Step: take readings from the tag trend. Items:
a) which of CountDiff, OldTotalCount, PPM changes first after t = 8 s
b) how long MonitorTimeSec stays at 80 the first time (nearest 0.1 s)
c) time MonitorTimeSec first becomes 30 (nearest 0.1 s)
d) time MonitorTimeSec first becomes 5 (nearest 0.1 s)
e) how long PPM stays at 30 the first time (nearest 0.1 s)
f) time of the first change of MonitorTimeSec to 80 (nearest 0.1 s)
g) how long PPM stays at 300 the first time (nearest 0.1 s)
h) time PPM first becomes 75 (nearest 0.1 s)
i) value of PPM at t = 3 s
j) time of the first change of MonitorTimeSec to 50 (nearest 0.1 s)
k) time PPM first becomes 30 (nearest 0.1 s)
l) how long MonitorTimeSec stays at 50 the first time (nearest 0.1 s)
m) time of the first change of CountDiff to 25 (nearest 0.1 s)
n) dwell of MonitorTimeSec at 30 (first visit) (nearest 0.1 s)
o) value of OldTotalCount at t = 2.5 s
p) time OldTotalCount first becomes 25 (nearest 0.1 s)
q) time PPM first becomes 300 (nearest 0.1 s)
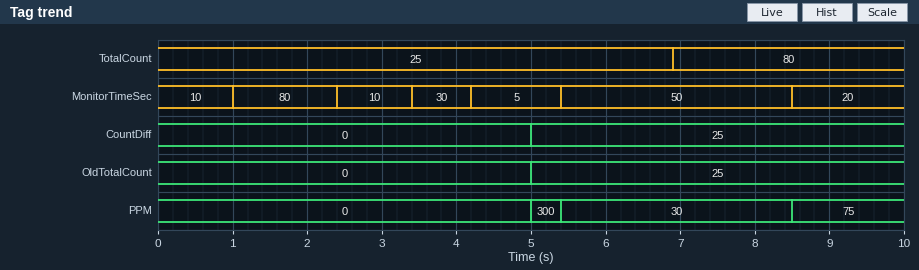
PPM
1.4 s
3.4 s
4.2 s
3.1 s
1.0 s
0.4 s
8.5 s
0
5.4 s
5.4 s
3.1 s
5.0 s
0.8 s
0
5.0 s
5.0 s
